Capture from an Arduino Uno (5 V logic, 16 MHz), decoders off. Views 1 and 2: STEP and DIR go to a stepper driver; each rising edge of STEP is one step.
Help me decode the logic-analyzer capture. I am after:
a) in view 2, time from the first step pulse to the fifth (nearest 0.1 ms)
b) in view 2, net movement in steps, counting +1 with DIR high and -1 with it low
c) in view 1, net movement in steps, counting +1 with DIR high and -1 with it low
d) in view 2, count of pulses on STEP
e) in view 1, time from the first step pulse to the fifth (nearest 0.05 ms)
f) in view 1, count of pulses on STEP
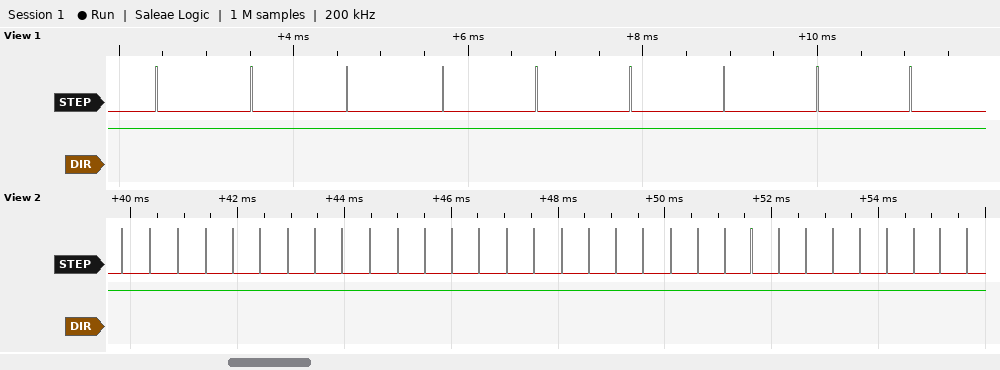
2.1 ms
+32
+9
32
4.35 ms
9
